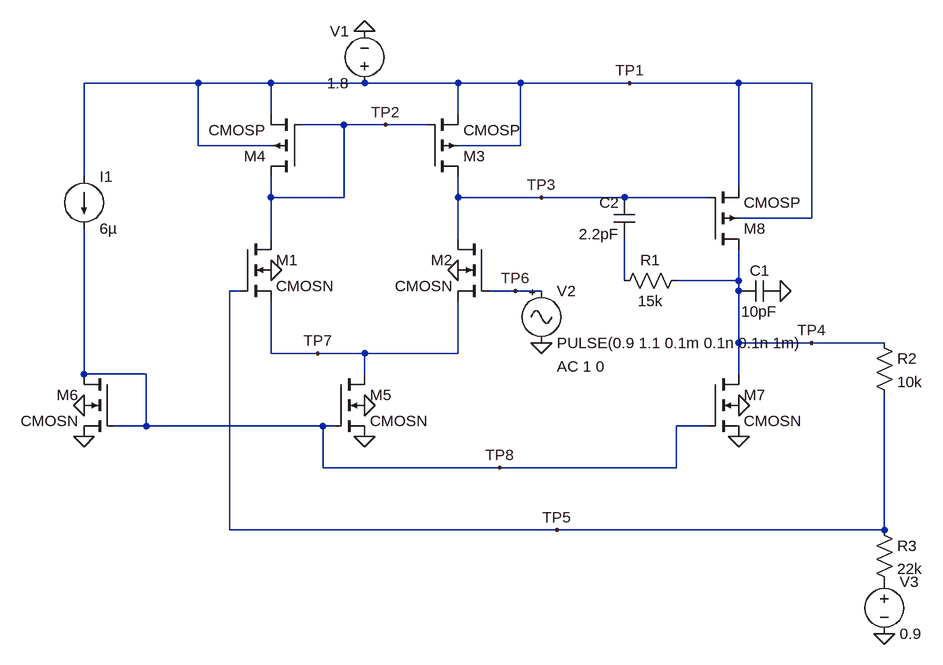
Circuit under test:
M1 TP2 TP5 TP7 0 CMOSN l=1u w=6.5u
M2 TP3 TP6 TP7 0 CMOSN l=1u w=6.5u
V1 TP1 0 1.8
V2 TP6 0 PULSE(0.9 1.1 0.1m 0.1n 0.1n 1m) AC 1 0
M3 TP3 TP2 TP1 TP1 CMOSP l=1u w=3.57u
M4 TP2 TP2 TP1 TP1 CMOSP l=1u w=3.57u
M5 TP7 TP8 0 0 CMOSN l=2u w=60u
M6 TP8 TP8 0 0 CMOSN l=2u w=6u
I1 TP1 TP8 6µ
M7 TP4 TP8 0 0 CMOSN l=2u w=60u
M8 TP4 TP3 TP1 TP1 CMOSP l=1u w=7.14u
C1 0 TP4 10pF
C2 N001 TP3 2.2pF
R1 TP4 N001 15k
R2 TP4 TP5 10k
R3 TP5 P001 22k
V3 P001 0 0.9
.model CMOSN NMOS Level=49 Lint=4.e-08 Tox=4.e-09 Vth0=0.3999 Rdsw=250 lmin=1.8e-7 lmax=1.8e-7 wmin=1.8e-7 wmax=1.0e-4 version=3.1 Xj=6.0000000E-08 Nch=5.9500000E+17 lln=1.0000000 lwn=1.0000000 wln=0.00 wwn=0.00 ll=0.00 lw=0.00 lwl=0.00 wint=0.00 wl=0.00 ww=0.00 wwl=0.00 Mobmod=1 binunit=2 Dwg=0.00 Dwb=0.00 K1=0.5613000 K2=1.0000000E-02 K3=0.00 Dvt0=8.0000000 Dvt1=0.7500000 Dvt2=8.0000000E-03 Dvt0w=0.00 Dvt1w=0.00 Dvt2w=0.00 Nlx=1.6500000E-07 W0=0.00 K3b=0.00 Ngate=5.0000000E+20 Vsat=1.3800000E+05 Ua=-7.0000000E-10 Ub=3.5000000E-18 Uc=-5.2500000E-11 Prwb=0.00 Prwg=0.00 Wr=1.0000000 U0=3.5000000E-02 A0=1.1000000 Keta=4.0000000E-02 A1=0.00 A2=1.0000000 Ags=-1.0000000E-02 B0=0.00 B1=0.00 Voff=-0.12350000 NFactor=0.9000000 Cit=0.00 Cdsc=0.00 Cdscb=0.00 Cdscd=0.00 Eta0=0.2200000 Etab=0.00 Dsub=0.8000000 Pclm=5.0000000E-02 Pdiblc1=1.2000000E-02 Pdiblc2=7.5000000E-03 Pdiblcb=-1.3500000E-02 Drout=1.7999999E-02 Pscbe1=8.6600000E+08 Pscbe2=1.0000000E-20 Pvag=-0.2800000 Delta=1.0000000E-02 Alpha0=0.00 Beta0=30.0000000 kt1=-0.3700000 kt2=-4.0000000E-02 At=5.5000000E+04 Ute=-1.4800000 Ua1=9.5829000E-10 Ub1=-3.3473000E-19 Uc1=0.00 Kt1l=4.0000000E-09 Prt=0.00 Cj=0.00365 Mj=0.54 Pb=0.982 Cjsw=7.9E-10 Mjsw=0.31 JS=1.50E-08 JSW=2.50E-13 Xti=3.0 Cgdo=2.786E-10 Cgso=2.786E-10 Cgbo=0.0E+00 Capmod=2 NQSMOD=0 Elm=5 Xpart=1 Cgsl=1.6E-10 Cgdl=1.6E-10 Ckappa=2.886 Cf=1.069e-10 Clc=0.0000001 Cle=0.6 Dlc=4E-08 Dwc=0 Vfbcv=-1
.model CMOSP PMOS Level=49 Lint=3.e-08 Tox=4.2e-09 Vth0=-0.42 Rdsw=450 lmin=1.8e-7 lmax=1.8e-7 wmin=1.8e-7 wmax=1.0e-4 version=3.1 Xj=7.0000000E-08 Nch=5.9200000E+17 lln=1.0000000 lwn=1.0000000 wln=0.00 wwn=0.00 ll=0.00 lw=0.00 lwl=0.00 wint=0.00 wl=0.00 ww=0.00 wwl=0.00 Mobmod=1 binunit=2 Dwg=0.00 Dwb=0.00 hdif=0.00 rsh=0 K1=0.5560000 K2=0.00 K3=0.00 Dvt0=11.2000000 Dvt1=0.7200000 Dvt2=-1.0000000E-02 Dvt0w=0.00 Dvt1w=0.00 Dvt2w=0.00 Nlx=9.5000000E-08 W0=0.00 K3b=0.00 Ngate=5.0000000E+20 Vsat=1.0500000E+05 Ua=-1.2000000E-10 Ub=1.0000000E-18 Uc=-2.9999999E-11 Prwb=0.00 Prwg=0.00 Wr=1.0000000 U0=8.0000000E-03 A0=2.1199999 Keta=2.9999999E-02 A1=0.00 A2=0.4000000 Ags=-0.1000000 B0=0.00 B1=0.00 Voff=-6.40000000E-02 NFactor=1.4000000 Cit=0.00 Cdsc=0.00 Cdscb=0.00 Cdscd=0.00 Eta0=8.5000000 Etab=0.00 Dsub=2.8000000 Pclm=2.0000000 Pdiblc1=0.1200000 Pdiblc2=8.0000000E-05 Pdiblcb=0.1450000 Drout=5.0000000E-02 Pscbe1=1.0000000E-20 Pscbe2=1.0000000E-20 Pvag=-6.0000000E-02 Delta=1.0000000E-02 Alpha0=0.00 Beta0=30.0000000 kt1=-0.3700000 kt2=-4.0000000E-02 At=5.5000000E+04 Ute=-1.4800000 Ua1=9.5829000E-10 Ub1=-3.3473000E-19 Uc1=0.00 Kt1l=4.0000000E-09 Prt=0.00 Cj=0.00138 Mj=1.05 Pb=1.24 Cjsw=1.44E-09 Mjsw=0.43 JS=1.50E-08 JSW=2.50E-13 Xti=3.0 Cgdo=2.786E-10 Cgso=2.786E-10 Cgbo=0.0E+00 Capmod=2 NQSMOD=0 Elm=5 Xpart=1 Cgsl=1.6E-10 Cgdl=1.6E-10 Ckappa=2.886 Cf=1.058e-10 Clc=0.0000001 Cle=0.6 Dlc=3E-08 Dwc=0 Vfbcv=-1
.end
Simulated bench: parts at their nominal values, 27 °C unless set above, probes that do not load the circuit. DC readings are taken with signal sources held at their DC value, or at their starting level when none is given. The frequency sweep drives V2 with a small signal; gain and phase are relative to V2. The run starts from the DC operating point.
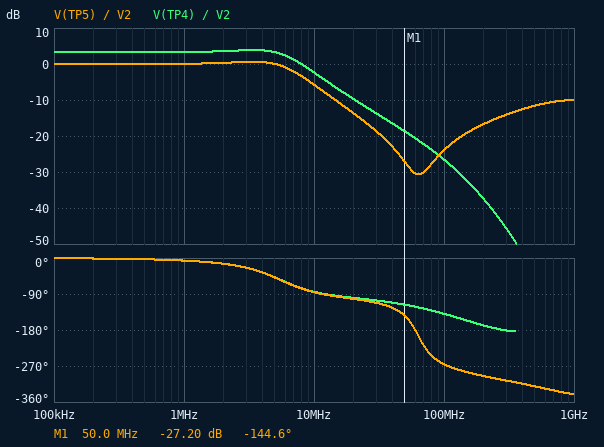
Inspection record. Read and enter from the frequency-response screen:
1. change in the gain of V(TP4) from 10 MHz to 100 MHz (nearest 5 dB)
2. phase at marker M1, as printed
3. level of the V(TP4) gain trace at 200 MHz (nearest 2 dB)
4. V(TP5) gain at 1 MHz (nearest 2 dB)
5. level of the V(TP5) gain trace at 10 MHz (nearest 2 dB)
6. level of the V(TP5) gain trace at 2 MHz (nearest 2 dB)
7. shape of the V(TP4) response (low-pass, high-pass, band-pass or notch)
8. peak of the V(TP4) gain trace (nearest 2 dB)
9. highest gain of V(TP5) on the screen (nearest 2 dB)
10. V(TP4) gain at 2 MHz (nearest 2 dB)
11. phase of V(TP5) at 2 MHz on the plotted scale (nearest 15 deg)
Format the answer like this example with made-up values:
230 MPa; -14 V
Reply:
-25 dB; -144.6 deg; -38 dB; 0 dB; -6 dB; 0 dB; low-pass; 4 dB; 0 dB; 4 dB; -15 deg
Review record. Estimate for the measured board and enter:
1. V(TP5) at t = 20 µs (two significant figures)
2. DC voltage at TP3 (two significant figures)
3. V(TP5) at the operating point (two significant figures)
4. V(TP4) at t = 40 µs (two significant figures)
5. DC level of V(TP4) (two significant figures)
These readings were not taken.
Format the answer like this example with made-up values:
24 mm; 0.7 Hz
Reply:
900 mV; 730 mV; 900 mV; 900 mV; 900 mV
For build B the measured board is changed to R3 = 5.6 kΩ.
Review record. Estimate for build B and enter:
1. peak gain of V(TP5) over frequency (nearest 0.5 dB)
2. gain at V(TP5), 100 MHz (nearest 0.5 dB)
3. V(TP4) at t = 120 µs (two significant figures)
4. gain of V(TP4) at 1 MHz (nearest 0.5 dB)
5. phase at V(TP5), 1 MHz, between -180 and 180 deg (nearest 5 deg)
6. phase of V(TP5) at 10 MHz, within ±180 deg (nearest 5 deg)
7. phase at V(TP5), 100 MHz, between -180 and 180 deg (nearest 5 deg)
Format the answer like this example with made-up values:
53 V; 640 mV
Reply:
0 dB; -29.5 dB; 1.4 V; 8.5 dB; -15 deg; -95 deg; 100 deg
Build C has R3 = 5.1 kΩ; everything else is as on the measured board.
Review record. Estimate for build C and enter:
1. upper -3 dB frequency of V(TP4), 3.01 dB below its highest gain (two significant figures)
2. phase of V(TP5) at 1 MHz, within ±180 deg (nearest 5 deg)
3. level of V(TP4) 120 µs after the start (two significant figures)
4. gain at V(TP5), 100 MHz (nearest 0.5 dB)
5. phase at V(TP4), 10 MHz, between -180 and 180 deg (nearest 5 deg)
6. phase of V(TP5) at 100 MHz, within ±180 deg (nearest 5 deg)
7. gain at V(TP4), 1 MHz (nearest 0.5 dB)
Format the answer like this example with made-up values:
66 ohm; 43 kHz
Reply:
4.3 MHz; -15 deg; 1.4 V; -30.0 dB; -95 deg; 100 deg; 9.0 dB
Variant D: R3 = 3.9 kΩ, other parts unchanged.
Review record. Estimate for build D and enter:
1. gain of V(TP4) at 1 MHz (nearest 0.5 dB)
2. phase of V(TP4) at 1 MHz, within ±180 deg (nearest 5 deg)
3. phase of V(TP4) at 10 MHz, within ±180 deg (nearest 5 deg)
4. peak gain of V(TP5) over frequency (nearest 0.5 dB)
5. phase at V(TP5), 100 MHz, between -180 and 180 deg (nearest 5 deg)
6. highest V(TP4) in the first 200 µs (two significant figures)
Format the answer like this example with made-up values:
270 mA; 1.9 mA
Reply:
10.5 dB; -20 deg; -100 deg; -0.5 dB; 100 deg; 1.4 V
